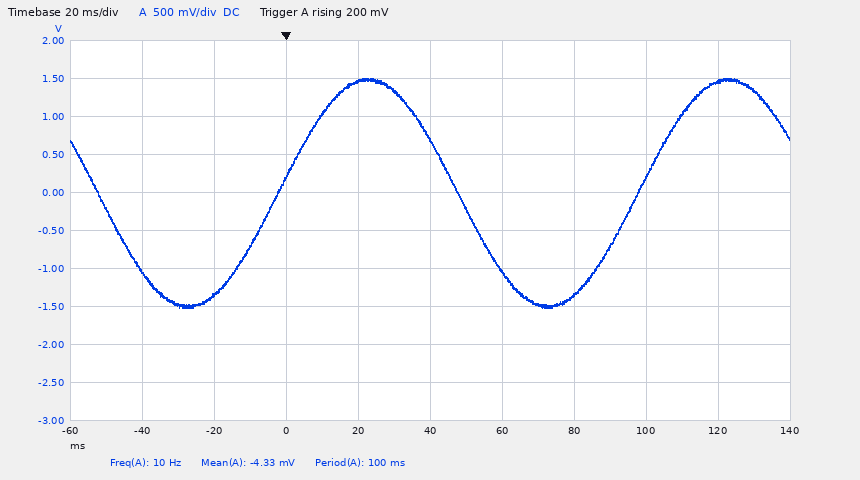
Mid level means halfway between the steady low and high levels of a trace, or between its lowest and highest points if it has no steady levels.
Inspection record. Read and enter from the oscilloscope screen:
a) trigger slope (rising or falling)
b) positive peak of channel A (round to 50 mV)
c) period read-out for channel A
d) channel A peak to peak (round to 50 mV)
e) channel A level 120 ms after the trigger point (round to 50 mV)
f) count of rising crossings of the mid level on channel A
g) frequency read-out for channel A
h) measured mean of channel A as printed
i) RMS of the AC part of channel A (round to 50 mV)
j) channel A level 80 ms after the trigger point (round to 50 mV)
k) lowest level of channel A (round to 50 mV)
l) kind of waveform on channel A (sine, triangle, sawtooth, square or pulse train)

rising
1.50 V
100 ms
3.00 V
1.45 V
2
10 Hz
-4.33 mV
1.05 V
-1.35 V
-1.50 V
sine
